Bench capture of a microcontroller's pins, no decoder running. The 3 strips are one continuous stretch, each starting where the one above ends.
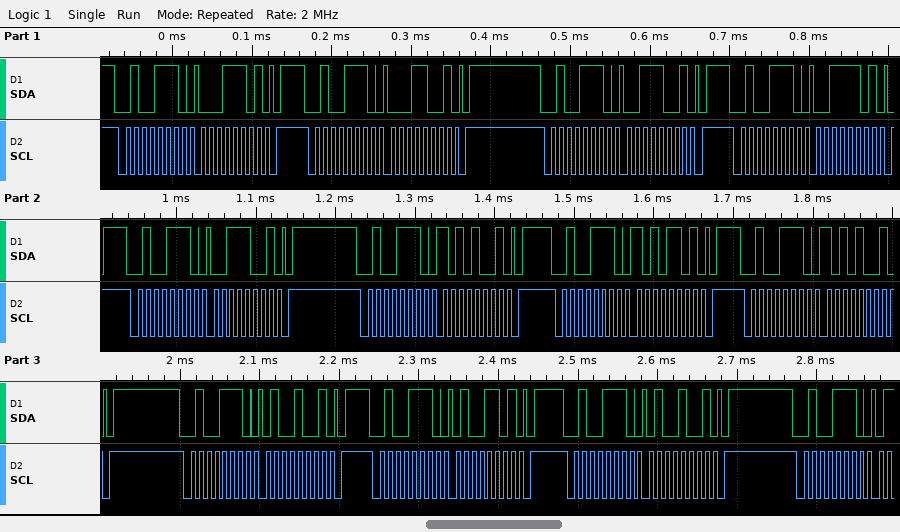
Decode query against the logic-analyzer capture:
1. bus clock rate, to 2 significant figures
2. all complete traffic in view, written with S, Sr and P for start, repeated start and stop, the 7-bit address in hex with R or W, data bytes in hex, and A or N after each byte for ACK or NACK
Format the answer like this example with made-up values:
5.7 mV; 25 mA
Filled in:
100 kHz; S 27W A 1D A P S 27W A 19 A P S 27W A 39 A P S 27W A 3D A P S 27W A 39 A P S 27W A A9 A P S 27W A AD A P S 27W A A9 A P S 27W A 49 A P S 27W A 4D A P S 27W A 49 A P S 27W A
